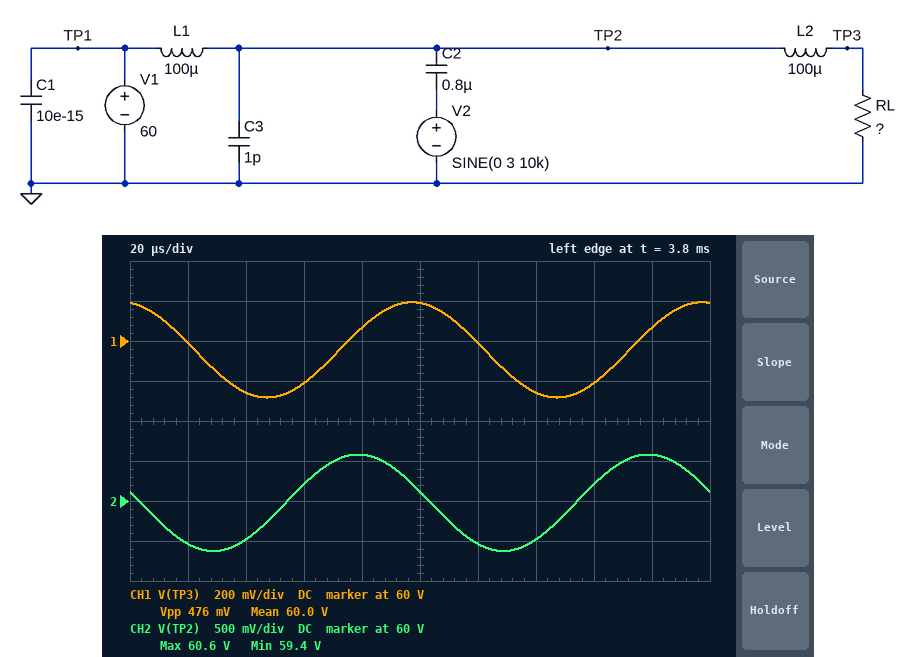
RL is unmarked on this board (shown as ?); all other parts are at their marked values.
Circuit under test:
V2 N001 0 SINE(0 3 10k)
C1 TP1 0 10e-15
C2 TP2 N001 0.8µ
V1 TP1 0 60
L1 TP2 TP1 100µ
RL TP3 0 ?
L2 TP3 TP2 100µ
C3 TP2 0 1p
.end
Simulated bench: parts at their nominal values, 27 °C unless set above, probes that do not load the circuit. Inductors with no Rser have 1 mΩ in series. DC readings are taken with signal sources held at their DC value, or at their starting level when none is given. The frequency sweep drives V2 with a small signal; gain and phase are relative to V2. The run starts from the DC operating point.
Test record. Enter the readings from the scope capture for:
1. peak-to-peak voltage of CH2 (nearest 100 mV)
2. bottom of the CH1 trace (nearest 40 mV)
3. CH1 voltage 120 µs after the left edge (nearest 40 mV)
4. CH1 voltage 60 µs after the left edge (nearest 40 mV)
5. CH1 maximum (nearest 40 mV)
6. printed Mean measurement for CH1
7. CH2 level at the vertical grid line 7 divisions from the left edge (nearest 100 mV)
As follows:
1.2 V
59.72 V
60.00 V
59.80 V
60.20 V
60.0 V
59.5 V
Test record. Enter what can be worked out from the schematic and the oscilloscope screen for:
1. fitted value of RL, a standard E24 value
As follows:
2.7 Ω
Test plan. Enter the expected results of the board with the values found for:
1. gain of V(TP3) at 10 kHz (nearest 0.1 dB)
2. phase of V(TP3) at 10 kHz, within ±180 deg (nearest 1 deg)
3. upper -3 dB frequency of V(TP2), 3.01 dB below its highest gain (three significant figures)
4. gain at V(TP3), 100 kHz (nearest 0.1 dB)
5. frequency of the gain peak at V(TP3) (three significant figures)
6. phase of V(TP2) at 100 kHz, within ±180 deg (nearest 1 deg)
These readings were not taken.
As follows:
-22.0 dB
100 deg
26.3 kHz
-26.8 dB
25.1 kHz
0 deg
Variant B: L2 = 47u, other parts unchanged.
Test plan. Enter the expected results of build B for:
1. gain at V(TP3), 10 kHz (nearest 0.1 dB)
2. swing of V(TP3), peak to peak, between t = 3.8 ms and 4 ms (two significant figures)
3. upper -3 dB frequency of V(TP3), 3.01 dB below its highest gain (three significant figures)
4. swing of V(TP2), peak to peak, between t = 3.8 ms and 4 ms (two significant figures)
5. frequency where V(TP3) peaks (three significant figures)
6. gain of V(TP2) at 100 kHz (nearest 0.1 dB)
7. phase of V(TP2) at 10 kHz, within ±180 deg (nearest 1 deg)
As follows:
-20.0 dB
600 mV
34.4 kHz
890 mV
31.2 kHz
0.9 dB
150 deg
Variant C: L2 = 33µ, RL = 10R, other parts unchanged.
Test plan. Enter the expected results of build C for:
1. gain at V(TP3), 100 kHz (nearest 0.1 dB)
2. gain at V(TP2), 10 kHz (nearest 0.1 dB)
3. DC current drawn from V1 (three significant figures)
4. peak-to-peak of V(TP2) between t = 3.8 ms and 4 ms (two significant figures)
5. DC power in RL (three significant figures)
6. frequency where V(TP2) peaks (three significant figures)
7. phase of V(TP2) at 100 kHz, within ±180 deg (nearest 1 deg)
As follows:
-6.2 dB
-10.1 dB
6.00 A
1.9 V
360 W
31.4 kHz
2 deg
